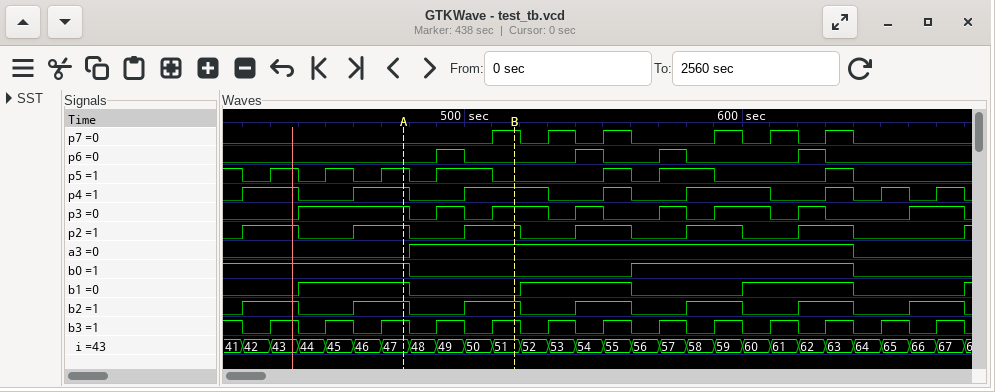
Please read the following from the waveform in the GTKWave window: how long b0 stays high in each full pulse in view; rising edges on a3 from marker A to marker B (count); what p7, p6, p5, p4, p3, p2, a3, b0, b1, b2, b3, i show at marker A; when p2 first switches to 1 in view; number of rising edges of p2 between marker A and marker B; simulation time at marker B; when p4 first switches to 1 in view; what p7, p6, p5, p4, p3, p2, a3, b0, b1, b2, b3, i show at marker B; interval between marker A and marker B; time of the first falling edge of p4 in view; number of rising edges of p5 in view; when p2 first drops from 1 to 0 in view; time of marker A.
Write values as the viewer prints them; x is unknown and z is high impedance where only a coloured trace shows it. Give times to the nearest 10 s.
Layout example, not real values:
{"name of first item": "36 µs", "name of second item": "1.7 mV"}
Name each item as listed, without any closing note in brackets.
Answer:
{"how long b0 stays high in each full pulse in view": "80 s", "rising edges on a3 from marker A to marker B": "1", "what p7, p6, p5, p4, p3, p2, a3, b0, b1, b2, b3, i show at marker A": "p7=0, p6=0, p5=1, p4=1, p3=1, p2=1, a3=0, b0=1, b1=1, b2=1, b3=1, i=47", "when p2 first switches to 1 in view": "420 s", "number of rising edges of p2 between marker A and marker B": "1", "simulation time at marker B": "520 s", "when p4 first switches to 1 in view": "420 s", "what p7, p6, p5, p4, p3, p2, a3, b0, b1, b2, b3, i show at marker B": "p7=1, p6=0, p5=0, p4=1, p3=1, p2=1, a3=1, b0=0, b1=0, b2=1, b3=1, i=51", "interval between marker A and marker B": "40 s", "time of the first falling edge of p4 in view": "440 s", "number of rising edges of p5 in view": "7", "when p2 first drops from 1 to 0 in view": "440 s", "time of marker A": "480 s"}
